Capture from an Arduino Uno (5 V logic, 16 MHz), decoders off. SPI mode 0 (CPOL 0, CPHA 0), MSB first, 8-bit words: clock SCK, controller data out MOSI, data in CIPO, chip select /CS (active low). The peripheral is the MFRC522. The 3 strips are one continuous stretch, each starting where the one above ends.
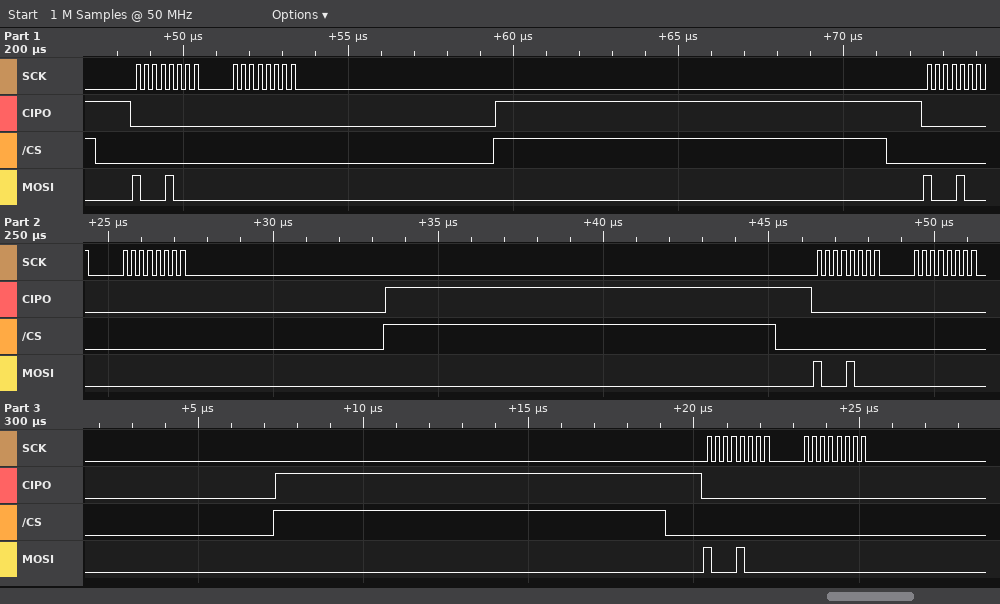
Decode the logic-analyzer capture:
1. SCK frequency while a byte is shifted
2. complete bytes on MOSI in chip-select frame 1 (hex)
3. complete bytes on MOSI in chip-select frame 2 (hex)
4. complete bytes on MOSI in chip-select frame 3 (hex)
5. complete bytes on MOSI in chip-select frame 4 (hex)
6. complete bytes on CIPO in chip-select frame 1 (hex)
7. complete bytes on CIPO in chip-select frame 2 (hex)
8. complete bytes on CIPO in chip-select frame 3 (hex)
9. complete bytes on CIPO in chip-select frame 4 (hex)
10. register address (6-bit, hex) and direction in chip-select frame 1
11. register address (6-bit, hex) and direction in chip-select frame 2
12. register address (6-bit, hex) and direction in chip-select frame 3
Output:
4 MHz
0x88 0x00
0x88 0x00
0x88 0x00
0x88 0x00
0x00 0x00
0x00 0x00
0x00 0x00
0x00 0x00
0x04 read
0x04 read
0x04 read
